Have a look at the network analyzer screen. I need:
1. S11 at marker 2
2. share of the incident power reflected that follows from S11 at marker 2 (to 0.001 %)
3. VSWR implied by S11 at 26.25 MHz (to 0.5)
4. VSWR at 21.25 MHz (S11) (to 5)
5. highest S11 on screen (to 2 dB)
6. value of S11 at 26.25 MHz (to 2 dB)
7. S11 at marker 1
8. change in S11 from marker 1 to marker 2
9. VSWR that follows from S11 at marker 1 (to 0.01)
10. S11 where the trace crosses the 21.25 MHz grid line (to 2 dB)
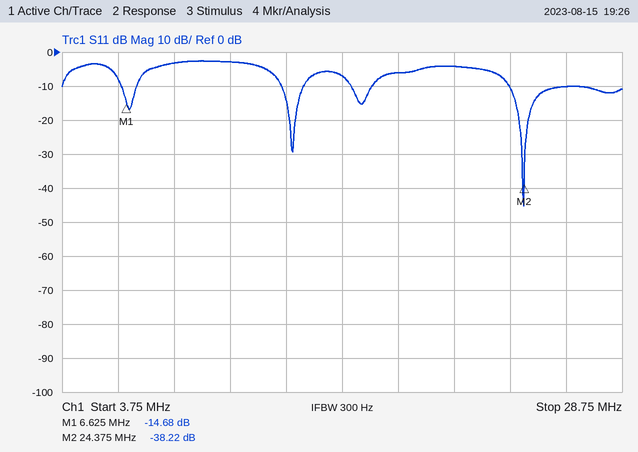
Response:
-38.22 dB
0.015 %
2.0
5
-2 dB
-10 dB
-14.68 dB
-23.54 dB
1.45
-4 dB
